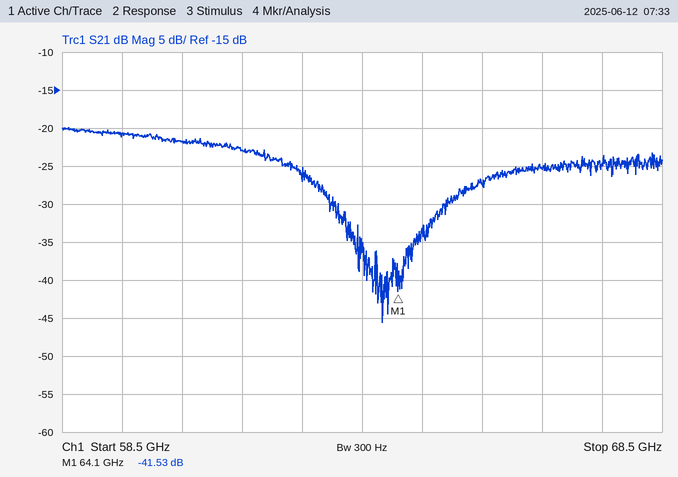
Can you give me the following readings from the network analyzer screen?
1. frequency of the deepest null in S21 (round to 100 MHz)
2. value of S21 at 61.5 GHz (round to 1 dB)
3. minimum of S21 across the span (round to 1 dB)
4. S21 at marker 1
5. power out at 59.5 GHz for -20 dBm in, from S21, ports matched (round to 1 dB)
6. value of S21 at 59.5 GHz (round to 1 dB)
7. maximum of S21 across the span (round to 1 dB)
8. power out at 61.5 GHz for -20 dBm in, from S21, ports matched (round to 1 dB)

63.8 GHz
-23 dB
-46 dB
-41.53 dB
-41 dBm
-21 dB
-20 dB
-43 dBm
